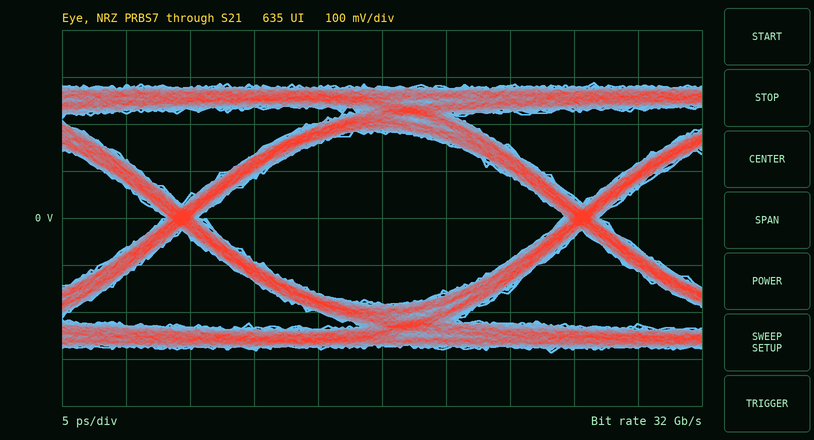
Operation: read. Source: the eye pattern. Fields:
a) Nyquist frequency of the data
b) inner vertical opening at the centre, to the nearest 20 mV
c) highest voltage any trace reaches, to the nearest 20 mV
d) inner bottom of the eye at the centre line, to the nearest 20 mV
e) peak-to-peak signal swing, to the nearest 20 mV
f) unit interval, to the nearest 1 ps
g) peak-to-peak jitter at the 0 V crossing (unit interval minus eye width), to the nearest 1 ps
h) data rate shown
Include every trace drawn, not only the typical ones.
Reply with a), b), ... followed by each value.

a) 16 GHz
b) 360 mV
c) 280 mV
d) -180 mV
e) 580 mV
f) 31 ps
g) 3 ps
h) 32 Gb/s
